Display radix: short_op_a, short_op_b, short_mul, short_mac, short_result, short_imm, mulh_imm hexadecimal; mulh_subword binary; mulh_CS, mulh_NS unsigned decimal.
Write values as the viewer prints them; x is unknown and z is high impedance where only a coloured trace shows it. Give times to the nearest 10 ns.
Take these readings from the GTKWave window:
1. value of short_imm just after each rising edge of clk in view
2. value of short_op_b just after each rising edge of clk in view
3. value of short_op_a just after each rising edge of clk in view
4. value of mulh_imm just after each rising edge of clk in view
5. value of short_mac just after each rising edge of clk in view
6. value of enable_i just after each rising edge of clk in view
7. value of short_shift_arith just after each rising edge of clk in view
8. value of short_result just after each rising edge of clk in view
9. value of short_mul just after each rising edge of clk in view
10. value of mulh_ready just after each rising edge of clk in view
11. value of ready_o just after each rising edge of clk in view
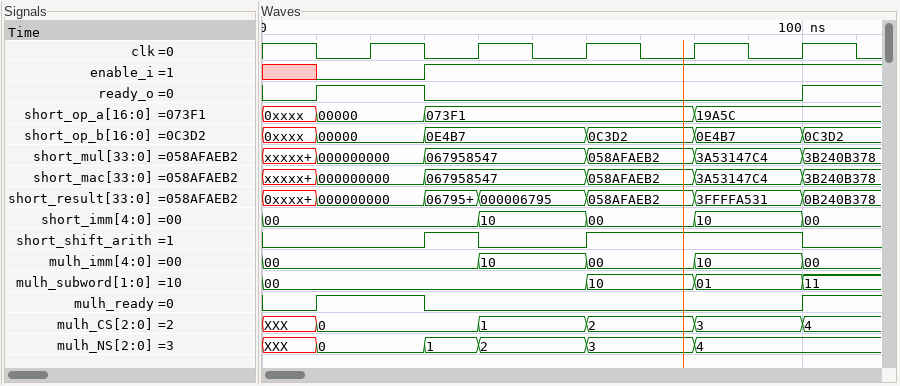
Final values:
00, 10, 00, 10, 00
00000, 0E4B7, 0C3D2, 0E4B7, 0C3D2
00000, 073F1, 073F1, 19A5C, 19A5C
00, 10, 00, 10, 00
000000000, 067958547, 058AFAEB2, 3A53147C4, 3B240B378
0 1 1 1 1
0 0 1 1 0
000000000, 000006795, 058AFAEB2, 3FFFFA531, 0B240B378
000000000, 067958547, 058AFAEB2, 3A53147C4, 3B240B378
1 0 0 0 1
1 0 0 0 1
